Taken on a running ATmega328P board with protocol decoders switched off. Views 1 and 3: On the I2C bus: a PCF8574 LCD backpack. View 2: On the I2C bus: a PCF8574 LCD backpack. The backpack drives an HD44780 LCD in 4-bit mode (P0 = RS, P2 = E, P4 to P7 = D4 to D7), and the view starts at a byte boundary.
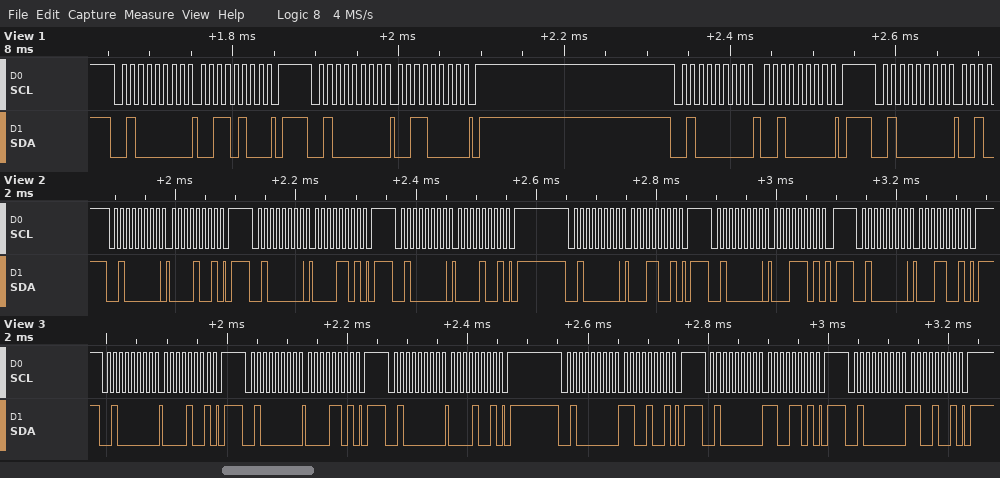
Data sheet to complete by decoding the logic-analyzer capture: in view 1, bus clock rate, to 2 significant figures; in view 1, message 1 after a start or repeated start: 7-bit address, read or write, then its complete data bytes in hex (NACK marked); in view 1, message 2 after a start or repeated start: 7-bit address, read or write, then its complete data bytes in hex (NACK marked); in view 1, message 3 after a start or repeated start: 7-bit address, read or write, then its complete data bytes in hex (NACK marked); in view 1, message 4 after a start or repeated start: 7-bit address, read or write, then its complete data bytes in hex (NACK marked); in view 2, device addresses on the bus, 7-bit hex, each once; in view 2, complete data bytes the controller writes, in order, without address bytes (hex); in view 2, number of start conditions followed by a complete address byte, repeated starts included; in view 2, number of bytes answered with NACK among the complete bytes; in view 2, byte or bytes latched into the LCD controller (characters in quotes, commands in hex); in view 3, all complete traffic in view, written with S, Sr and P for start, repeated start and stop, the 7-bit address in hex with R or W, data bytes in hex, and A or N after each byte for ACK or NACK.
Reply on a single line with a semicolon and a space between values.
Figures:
100 kHz; 0x20 write: 34; 0x20 write: 30; 0x20 write: 20; 0x20 write; 0x20; 09 0D 09 19 1D 19; 6; 0; data 0x01; S 20W A 09 A P S 20W A 0D A P S 20W A 09 A P S 20W A C9 A P S 20W A CD A P S 20W A C9 A P
